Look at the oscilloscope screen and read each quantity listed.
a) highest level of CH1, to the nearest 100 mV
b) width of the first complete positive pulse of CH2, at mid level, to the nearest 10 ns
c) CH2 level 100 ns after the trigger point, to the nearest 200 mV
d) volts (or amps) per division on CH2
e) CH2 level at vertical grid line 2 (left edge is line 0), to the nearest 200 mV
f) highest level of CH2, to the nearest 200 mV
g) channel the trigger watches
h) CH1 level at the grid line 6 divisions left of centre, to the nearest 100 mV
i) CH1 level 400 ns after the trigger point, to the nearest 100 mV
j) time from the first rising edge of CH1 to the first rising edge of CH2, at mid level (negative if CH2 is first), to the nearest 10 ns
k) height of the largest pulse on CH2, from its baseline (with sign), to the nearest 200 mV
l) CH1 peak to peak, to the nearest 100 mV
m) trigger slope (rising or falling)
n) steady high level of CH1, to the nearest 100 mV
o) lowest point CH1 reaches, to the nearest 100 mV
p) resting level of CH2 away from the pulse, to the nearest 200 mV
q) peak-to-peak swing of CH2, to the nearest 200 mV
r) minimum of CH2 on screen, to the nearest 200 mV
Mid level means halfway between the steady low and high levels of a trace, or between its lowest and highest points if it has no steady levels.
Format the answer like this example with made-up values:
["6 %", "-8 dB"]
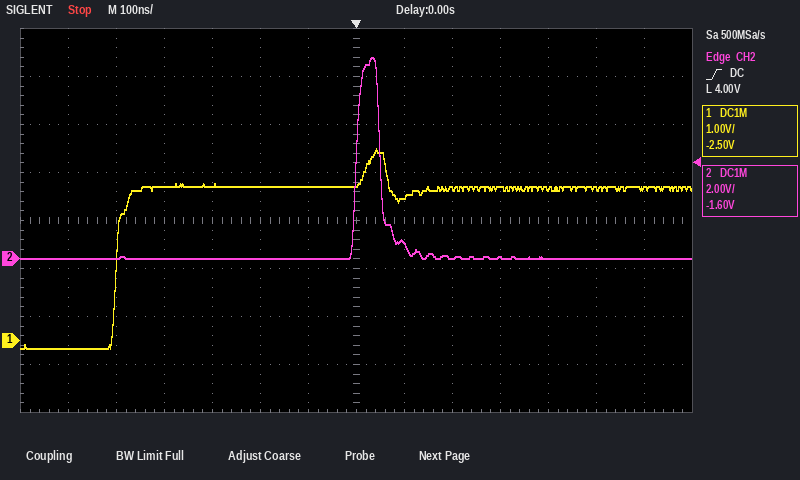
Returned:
["4.0 V", "50 ns", "600 mV", "2 V", "0.0 V", "8.4 V", "CH2", "-200 mV", "3.2 V", "+500 ns", "+8.4 V", "4.2 V", "rising", "3.2 V", "-200 mV", "0.0 V", "8.4 V", "0.0 V"]
